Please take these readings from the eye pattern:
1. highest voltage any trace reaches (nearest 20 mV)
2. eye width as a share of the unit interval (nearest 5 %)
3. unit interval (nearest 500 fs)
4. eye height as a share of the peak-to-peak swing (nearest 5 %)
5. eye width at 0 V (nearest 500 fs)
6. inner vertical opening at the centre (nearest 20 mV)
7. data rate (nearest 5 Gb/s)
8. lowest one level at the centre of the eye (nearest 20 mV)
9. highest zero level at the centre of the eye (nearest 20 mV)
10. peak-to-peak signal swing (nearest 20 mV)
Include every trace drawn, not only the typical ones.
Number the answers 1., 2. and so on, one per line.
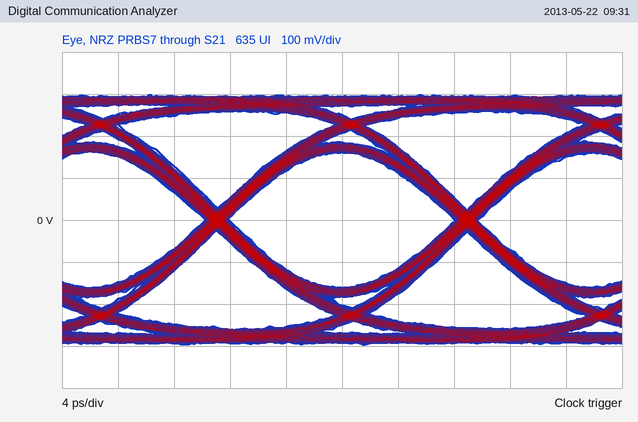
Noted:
1. 300 mV
2. 90 %
3. 18.0 ps
4. 55 %
5. 16.0 ps
6. 320 mV
7. 55 Gb/s
8. 160 mV
9. -160 mV
10. 600 mV
